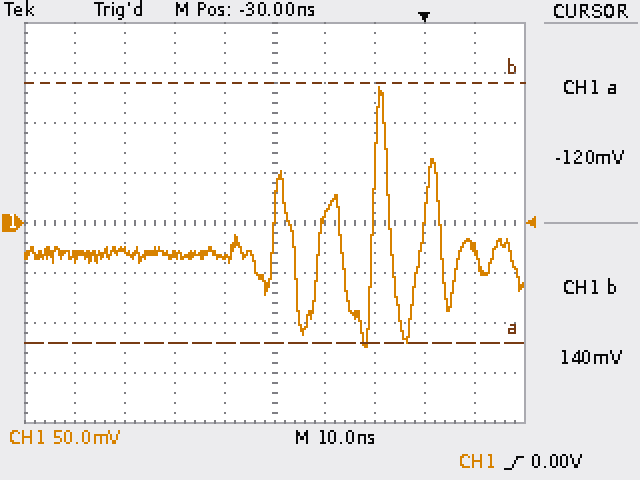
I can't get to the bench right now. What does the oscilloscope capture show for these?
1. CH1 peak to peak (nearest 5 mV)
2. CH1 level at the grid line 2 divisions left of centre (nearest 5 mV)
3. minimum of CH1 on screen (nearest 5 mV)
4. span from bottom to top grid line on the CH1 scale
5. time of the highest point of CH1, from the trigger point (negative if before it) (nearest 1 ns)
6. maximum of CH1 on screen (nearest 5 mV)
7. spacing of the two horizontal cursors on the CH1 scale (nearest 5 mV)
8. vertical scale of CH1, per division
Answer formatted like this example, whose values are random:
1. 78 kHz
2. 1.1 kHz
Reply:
1. 260 mV
2. -30 mV
3. -125 mV
4. 400 mV
5. -9 ns
6. 135 mV
7. 260 mV
8. 50 mV
